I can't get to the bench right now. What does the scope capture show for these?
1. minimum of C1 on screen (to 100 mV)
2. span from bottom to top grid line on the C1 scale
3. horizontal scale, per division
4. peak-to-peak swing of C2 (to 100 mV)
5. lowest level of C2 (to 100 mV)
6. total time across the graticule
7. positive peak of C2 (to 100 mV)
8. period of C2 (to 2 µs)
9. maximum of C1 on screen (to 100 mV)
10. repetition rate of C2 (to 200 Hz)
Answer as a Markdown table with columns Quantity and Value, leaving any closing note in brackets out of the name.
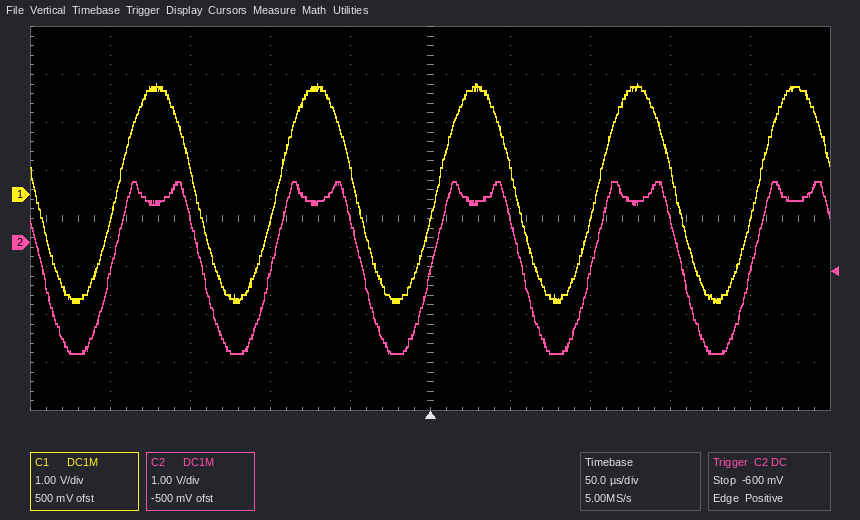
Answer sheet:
| Quantity | Value |
|---|---|
| minimum of C1 on screen | -2.2 V |
| span from bottom to top grid line on the C1 scale | 8 V |
| horizontal scale, per division | 50 µs |
| peak-to-peak swing of C2 | 3.6 V |
| lowest level of C2 | -2.3 V |
| total time across the graticule | 500 µs |
| positive peak of C2 | 1.3 V |
| period of C2 | 100 µs |
| maximum of C1 on screen | 2.3 V |
| repetition rate of C2 | 10.0 kHz |
